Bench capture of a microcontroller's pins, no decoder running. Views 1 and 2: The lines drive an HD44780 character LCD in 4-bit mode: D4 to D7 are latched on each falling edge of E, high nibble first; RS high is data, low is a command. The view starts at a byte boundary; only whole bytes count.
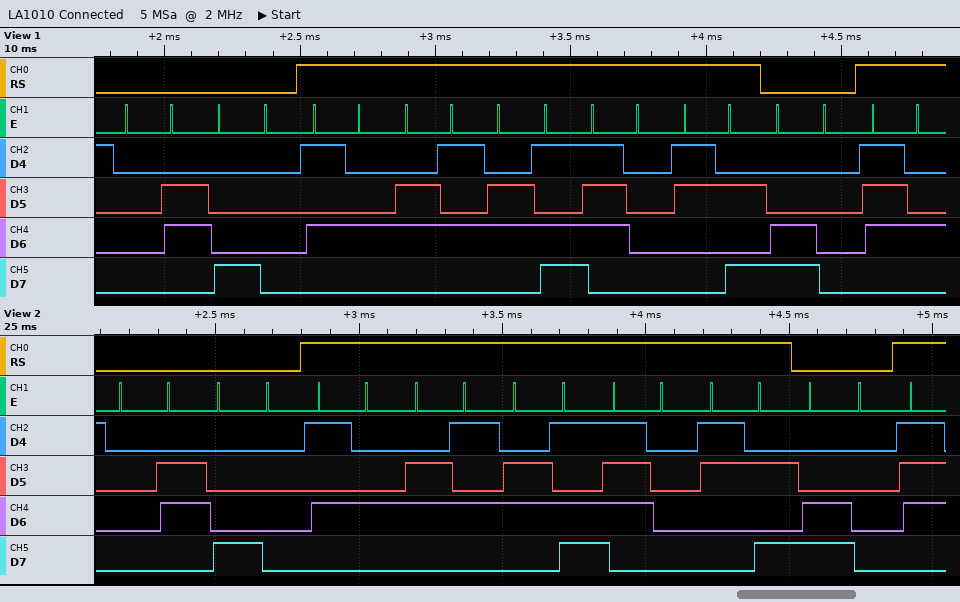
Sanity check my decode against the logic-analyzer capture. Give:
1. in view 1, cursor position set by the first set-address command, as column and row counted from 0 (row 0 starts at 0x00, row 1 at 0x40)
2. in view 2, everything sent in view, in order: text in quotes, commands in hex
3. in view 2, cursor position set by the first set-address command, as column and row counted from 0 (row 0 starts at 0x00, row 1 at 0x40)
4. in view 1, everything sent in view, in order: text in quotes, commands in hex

column 0, row 0
0x06 0x80 "Temp:" 0xC0
column 0, row 0
0x06 0x80 "Temp:" 0xC0 "t"
